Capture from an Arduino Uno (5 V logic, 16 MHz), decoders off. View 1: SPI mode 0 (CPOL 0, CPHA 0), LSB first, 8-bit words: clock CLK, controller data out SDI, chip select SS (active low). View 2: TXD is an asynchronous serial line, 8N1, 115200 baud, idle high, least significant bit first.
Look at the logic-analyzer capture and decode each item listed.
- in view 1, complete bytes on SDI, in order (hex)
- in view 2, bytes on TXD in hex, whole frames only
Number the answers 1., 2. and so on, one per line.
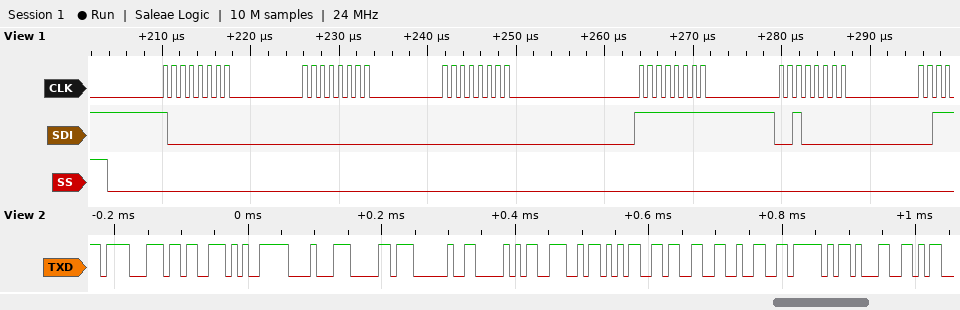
1. 01 00 00 FF 04
2. 8F 9B E5 88 B0 20 50 4E 35 33 32 5F 31
